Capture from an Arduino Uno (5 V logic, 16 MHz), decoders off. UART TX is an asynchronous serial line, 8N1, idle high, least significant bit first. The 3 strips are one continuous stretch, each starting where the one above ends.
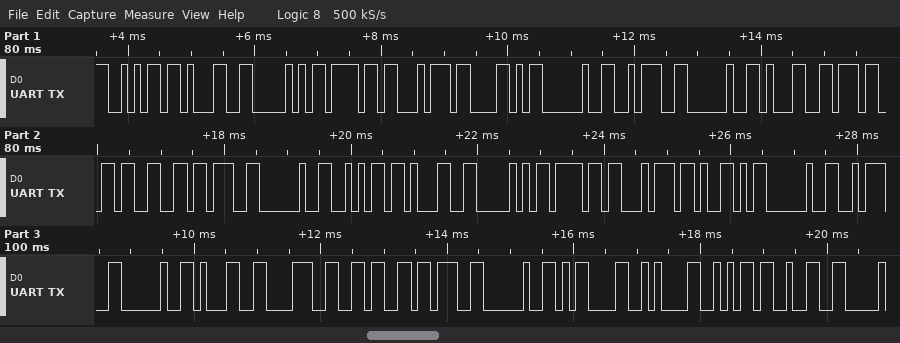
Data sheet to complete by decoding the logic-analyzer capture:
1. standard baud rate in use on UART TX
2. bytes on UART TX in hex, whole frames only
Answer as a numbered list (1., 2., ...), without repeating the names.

1. 9600 baud
2. 6A 31 50 6F 74 58 20 3A 20 31 37 33 3B 20 6A 31 50 6F 74 59 20 3A 20 31 38 36 3B 20 0D 0A 6A 32
